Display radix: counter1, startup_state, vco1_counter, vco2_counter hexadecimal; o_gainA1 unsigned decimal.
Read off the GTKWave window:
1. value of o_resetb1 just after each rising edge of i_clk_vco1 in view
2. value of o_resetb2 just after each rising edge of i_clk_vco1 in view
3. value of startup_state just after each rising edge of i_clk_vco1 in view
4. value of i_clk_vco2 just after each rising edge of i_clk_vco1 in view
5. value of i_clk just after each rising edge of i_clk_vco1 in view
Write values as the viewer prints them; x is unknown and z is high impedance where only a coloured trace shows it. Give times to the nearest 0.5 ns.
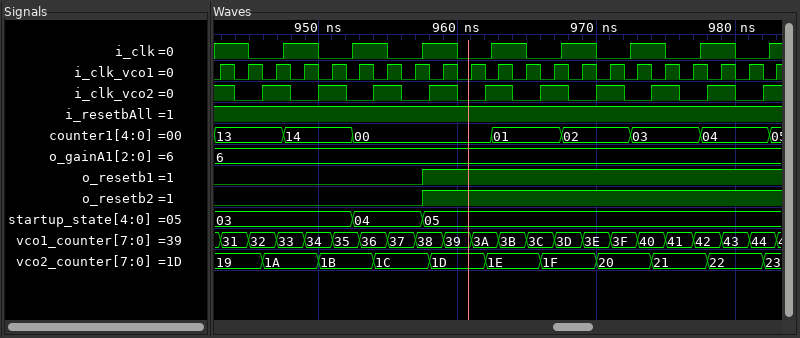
0 0 0 0 0 0 0 0 1 1 1 1 1 1 1 1 1 1 1 1 1
0 0 0 0 0 0 0 0 1 1 1 1 1 1 1 1 1 1 1 1 1
03, 03, 03, 03, 03, 04, 04, 04, 05, 05, 05, 05, 05, 05, 05, 05, 05, 05, 05, 05, 05
1 0 1 0 1 0 1 0 1 0 1 0 1 0 1 0 1 0 1 0 1
1 0 0 1 0 1 0 0 1 0 1 0 0 1 0 1 0 0 1 0 1
